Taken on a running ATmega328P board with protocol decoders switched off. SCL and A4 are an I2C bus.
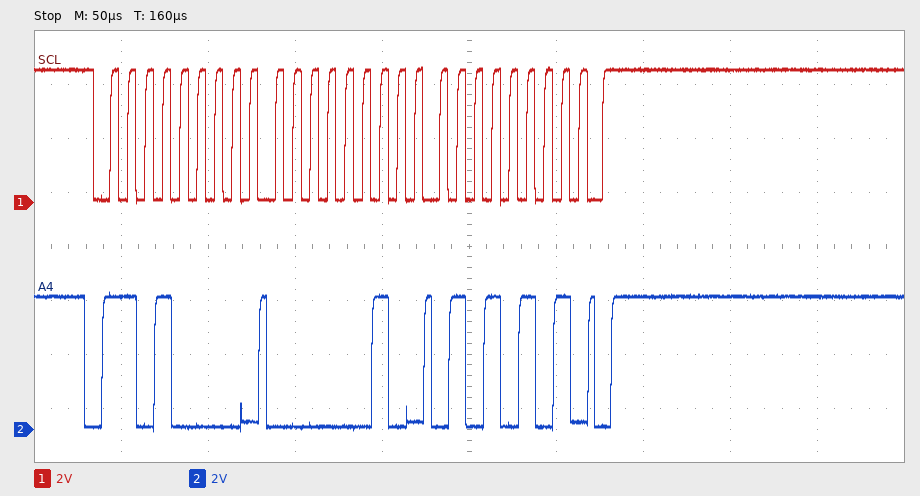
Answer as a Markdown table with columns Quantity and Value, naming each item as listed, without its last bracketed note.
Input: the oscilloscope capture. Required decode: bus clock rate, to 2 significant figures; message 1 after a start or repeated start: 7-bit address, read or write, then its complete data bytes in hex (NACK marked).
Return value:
| Quantity | Value |
|---|---|
| bus clock rate, to 2 significant figures | 100 kHz |
| message 1 after a start or repeated start: 7-bit address, read or write, then its complete data bytes in hex | 0x68 write: 02 55 |
